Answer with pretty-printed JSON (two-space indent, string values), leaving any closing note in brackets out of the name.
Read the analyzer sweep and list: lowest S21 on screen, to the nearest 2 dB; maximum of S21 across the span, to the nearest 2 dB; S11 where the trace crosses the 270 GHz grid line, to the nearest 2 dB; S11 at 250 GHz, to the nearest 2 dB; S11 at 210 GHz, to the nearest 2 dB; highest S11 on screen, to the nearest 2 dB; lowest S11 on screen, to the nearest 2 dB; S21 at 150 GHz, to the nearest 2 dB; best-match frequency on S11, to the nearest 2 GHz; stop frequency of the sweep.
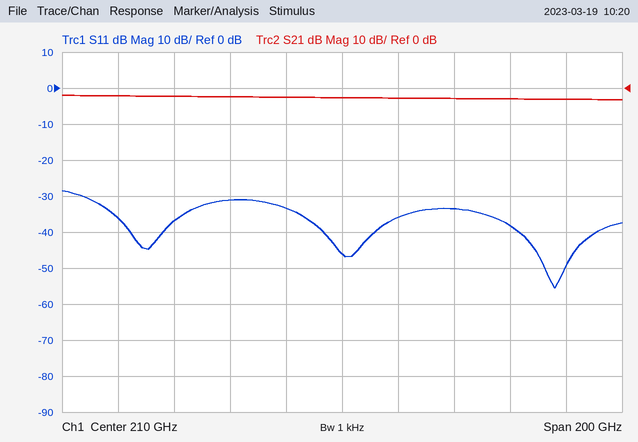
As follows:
{
  "lowest S21 on screen, to the nearest 2 dB": "-4 dB",
  "maximum of S21 across the span, to the nearest 2 dB": "-2 dB",
  "S11 where the trace crosses the 270 GHz grid line, to the nearest 2 dB": "-38 dB",
  "S11 at 250 GHz, to the nearest 2 dB": "-34 dB",
  "S11 at 210 GHz, to the nearest 2 dB": "-46 dB",
  "highest S11 on screen, to the nearest 2 dB": "-28 dB",
  "lowest S11 on screen, to the nearest 2 dB": "-56 dB",
  "S21 at 150 GHz, to the nearest 2 dB": "-2 dB",
  "best-match frequency on S11, to the nearest 2 GHz": "286 GHz",
  "stop frequency of the sweep": "310 GHz"
}
